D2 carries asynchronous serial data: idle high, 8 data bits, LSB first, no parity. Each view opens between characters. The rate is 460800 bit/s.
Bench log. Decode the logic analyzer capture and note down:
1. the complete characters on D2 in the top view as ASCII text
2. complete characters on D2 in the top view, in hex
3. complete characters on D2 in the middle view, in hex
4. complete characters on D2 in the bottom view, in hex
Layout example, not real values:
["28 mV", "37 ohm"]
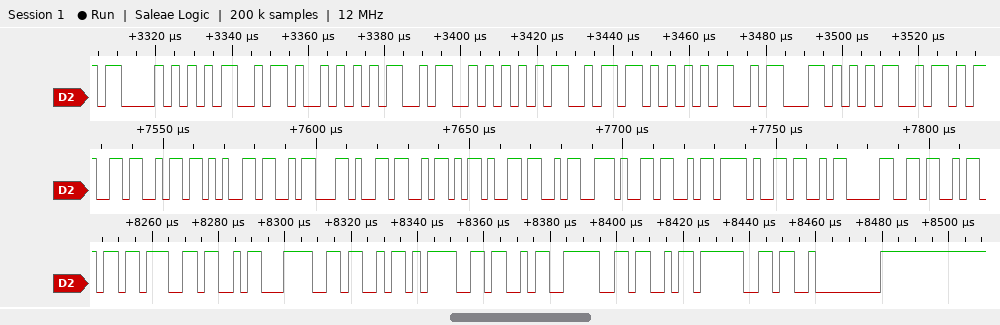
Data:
["\"C5K5S5[5c5\"", "43, 35, 4B, 35, 53, 35, 5B, 35, 63, 35", "36, 5B, 36, 63, 36, 6B, 36, 73, 36, 7B, 36, 83, 36", "DB, 36, E3, 36, EB, 36, F3, 36, FB, 36, 00"]
